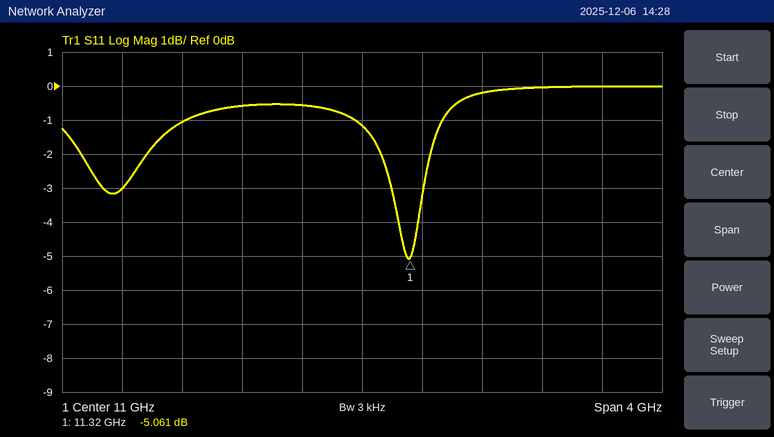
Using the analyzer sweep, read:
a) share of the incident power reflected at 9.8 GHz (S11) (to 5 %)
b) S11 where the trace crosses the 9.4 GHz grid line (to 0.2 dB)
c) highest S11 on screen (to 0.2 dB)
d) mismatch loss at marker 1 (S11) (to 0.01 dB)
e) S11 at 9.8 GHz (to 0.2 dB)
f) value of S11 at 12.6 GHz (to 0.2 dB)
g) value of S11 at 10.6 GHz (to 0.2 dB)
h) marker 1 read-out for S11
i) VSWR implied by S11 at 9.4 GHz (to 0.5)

80 %
-3.0 dB
0.0 dB
1.62 dB
-1.0 dB
0.0 dB
-0.6 dB
-5.061 dB
6.0
